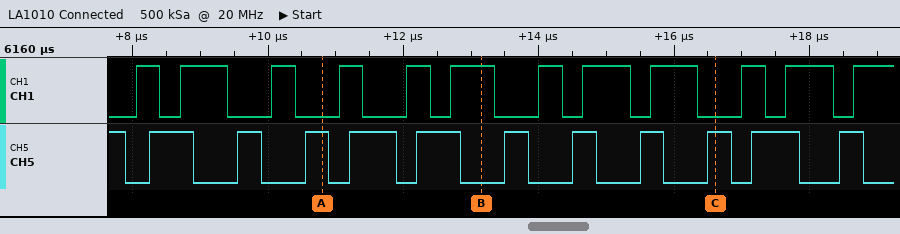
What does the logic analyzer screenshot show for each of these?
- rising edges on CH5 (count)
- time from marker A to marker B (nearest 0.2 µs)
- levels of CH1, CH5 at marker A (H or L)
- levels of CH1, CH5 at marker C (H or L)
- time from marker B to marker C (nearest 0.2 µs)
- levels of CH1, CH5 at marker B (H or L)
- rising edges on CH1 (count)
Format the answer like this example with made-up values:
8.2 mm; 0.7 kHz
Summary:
11; 2.4 µs; CH1=L, CH5=H; CH1=L, CH5=H; 3.4 µs; CH1=H, CH5=L; 12
